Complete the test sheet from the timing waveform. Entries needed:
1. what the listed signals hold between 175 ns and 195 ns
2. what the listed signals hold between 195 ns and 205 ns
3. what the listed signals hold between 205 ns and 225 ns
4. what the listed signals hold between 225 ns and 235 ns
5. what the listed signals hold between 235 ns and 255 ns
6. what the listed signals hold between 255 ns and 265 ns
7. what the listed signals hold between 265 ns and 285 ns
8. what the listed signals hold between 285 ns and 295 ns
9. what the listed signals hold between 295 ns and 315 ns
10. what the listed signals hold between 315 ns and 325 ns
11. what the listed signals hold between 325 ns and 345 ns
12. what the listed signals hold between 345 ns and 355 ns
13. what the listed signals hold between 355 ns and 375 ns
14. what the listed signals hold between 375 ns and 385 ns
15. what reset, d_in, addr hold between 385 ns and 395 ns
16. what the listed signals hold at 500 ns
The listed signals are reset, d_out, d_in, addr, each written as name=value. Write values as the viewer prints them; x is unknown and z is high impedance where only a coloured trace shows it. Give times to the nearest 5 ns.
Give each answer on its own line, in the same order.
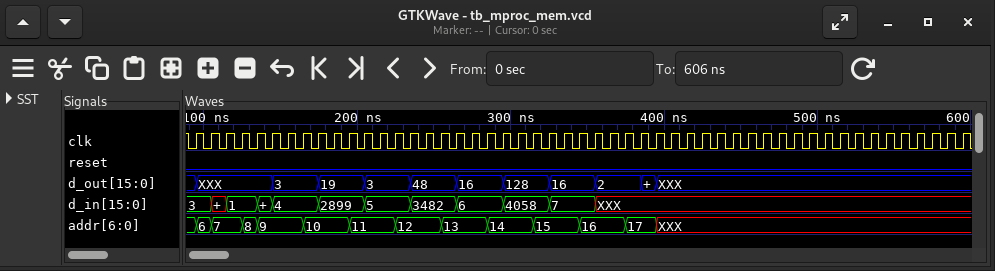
reset=0, d_out=19, d_in=2899, addr=10
reset=0, d_out=19, d_in=2899, addr=11
reset=0, d_out=3, d_in=5, addr=11
reset=0, d_out=3, d_in=5, addr=12
reset=0, d_out=48, d_in=3482, addr=12
reset=0, d_out=48, d_in=3482, addr=13
reset=0, d_out=16, d_in=6, addr=13
reset=0, d_out=16, d_in=6, addr=14
reset=0, d_out=128, d_in=4058, addr=14
reset=0, d_out=128, d_in=4058, addr=15
reset=0, d_out=16, d_in=7, addr=15
reset=0, d_out=16, d_in=7, addr=16
reset=0, d_out=2, d_in=XXX, addr=16
reset=0, d_out=2, d_in=XXX, addr=17
reset=0, d_in=XXX, addr=17
reset=0, d_out=XXX, d_in=XXX, addr=XXX
